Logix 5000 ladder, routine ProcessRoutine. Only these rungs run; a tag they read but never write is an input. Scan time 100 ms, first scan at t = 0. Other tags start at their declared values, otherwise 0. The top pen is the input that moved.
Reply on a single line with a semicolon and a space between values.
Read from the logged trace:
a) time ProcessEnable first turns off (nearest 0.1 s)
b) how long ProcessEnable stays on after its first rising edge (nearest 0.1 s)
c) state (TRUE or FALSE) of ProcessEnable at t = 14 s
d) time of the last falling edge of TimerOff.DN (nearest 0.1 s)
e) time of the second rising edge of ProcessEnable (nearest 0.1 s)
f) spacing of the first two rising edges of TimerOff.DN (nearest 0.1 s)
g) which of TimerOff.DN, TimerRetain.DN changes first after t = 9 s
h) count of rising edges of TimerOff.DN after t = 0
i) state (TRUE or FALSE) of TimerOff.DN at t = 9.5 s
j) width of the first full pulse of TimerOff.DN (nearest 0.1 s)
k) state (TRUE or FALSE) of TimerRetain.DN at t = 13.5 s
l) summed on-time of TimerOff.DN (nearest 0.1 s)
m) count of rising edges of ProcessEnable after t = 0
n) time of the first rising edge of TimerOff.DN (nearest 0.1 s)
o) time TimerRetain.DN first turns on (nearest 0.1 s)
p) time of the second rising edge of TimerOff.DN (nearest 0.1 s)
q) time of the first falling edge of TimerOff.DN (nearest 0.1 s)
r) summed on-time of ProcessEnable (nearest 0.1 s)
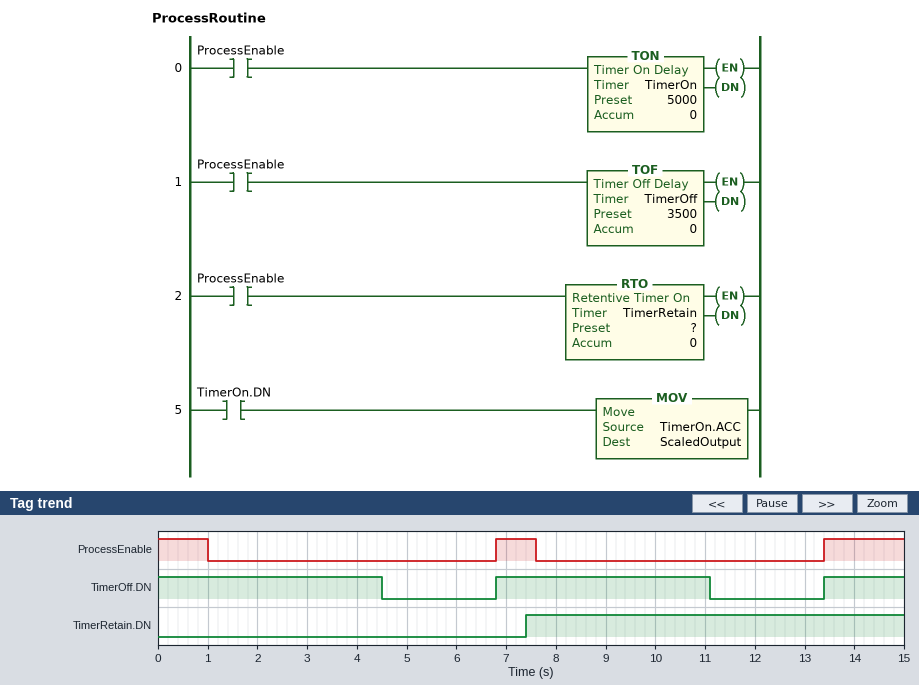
1.0 s; 0.8 s; TRUE; 11.1 s; 13.4 s; 6.6 s; TimerOff.DN; 2; TRUE; 4.3 s; TRUE; 10.4 s; 2; 6.8 s; 7.4 s; 13.4 s; 4.5 s; 3.4 s
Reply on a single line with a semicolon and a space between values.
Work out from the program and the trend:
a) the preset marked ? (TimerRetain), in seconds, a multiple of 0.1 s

1.5 s
